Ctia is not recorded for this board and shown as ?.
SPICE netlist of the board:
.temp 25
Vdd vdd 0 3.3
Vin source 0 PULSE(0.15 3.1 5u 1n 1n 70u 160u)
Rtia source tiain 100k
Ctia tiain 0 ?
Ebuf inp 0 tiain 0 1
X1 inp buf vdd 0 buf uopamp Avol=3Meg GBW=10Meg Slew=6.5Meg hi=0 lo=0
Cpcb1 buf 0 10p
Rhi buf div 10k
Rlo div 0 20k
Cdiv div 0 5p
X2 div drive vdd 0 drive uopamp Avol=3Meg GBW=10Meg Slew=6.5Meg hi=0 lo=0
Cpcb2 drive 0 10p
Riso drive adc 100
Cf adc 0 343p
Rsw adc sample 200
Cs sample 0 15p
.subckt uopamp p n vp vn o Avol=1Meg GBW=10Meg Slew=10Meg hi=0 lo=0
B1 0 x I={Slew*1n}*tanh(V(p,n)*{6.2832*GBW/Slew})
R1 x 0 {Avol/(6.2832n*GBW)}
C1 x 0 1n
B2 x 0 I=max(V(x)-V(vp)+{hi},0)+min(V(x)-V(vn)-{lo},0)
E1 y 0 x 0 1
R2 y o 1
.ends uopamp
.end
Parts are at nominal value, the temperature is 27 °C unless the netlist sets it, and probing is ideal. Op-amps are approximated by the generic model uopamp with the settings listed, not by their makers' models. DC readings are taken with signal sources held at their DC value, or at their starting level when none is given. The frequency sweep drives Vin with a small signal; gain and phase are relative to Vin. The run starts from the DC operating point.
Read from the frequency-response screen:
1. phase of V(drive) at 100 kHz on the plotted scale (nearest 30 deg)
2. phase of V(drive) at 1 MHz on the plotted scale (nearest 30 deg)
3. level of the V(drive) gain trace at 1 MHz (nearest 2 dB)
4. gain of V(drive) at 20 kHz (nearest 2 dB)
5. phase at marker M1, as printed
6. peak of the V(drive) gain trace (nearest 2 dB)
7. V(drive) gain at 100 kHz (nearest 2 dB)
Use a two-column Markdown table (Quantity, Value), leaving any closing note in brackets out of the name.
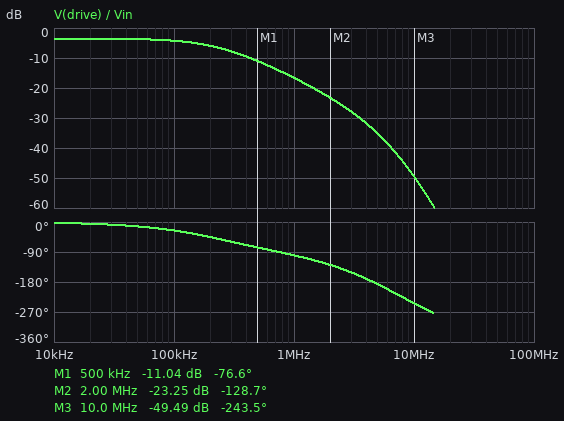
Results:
| Quantity | Value |
|---|---|
| phase of V(drive) at 100 kHz on the plotted scale | -30 deg |
| phase of V(drive) at 1 MHz on the plotted scale | -90 deg |
| level of the V(drive) gain trace at 1 MHz | -16 dB |
| gain of V(drive) at 20 kHz | -4 dB |
| phase at marker M1, as printed | -76.6 deg |
| peak of the V(drive) gain trace | -4 dB |
| V(drive) gain at 100 kHz | -4 dB |
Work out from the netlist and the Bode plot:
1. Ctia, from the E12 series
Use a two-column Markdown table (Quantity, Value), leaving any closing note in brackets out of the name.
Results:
| Quantity | Value |
|---|---|
| Ctia, from the E12 series | 6.8 pF |
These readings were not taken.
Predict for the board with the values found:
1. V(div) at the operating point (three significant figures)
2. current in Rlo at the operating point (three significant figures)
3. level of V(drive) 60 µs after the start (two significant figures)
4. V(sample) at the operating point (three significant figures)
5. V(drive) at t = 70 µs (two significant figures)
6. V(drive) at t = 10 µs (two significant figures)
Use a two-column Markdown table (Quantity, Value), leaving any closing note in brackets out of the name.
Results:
| Quantity | Value |
|---|---|
| V(div) at the operating point | 100 mV |
| current in Rlo at the operating point | 5.00 µA |
| level of V(drive) 60 µs after the start | 2.1 V |
| V(sample) at the operating point | 100 mV |
| V(drive) at t = 70 µs | 2.1 V |
| V(drive) at t = 10 µs | 2.1 V |
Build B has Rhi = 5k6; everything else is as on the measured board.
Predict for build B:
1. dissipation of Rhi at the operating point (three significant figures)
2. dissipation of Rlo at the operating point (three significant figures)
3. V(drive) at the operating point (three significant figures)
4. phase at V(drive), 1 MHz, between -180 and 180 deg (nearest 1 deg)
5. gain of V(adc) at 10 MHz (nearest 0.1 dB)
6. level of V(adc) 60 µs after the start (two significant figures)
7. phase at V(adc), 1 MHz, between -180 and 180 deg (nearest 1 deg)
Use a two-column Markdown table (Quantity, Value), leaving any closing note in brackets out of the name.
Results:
| Quantity | Value |
|---|---|
| dissipation of Rhi at the operating point | 192 nW |
| dissipation of Rlo at the operating point | 687 nW |
| V(drive) at the operating point | 117 mV |
| phase at V(drive), 1 MHz, between -180 and 180 deg | -96 deg |
| gain of V(adc) at 10 MHz | -53.2 dB |
| level of V(adc) 60 µs after the start | 2.4 V |
| phase at V(adc), 1 MHz, between -180 and 180 deg | -109 deg |
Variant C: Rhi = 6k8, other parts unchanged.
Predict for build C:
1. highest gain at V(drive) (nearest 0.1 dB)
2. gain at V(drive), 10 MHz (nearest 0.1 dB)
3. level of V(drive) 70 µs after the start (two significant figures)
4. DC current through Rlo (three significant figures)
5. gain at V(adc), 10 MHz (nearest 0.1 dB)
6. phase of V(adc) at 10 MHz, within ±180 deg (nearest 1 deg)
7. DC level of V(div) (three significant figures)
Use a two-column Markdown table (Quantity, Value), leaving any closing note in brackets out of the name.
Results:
| Quantity | Value |
|---|---|
| highest gain at V(drive) | -2.5 dB |
| gain at V(drive), 10 MHz | -46.7 dB |
| level of V(drive) 70 µs after the start | 2.3 V |
| DC current through Rlo | 5.60 µA |
| gain at V(adc), 10 MHz | -54.5 dB |
| phase of V(adc) at 10 MHz, within ±180 deg | 57 deg |
| DC level of V(div) | 112 mV |
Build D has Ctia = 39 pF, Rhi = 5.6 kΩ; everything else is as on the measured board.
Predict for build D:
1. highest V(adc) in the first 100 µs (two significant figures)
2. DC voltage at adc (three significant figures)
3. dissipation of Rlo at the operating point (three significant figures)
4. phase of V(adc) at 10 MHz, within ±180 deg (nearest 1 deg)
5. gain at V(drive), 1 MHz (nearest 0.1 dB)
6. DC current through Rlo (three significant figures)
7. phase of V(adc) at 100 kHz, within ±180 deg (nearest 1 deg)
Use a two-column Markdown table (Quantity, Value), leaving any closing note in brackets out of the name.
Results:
| Quantity | Value |
|---|---|
| highest V(adc) in the first 100 µs | 2.4 V |
| DC voltage at adc | 117 mV |
| dissipation of Rlo at the operating point | 687 nW |
| phase of V(adc) at 10 MHz, within ±180 deg | 60 deg |
| gain at V(drive), 1 MHz | -30.1 dB |
| DC current through Rlo | 5.86 µA |
| phase of V(adc) at 100 kHz, within ±180 deg | -71 deg |
